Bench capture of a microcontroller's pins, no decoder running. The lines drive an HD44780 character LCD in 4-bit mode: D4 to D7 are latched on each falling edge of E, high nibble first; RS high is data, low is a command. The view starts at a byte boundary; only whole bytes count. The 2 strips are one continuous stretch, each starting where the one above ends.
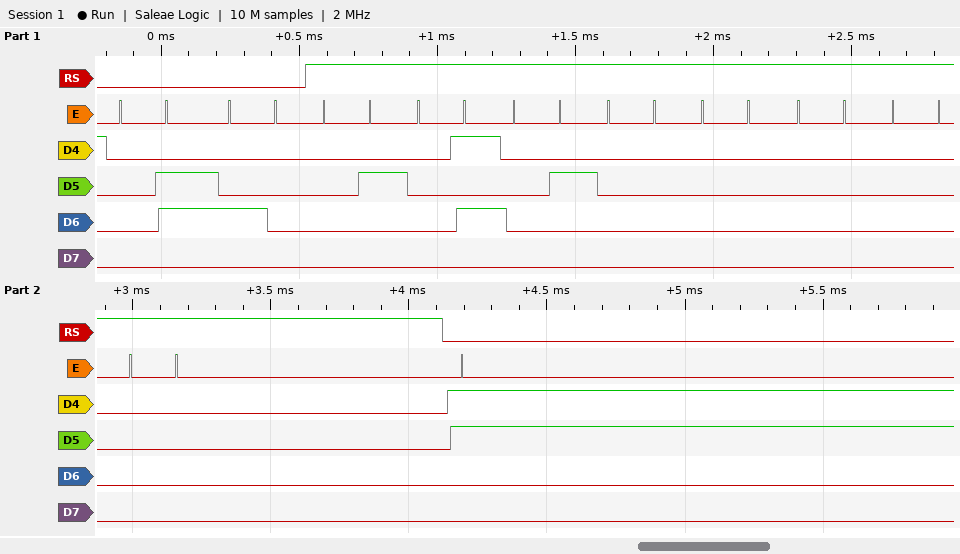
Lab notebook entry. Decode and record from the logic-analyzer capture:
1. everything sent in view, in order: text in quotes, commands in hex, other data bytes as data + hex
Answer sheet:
0x06 0x40 data 02 05 02 00 00 00 00 00
